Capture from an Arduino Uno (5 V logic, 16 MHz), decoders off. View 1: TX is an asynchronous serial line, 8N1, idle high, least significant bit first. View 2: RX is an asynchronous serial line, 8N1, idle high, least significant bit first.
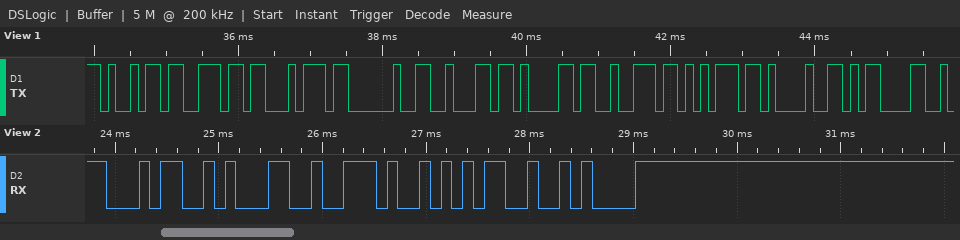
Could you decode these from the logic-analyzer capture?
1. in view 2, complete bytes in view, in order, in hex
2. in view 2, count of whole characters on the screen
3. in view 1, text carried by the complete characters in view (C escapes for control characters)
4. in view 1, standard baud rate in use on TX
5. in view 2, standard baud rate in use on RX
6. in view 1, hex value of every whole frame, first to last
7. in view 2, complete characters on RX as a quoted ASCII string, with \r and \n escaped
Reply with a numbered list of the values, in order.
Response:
1. 34 31 2E 35 0A
2. 5
3. "int baru!\r"
4. 9600 baud
5. 9600 baud
6. 69 6E 74 20 62 61 72 75 21 0D
7. "41.5\n"
